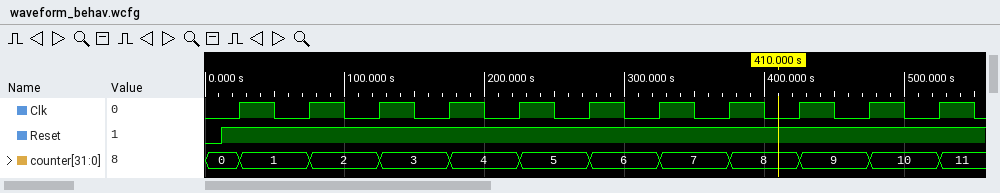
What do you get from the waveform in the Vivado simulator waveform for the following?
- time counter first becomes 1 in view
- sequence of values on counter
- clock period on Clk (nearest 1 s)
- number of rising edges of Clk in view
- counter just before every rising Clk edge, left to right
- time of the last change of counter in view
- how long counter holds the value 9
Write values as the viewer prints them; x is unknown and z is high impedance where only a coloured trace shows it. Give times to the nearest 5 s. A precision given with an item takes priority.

25 s
0, 1, 2, 3, 4, 5, 6, 7, 8, 9, 10, 11
50 s
11
0, 1, 2, 3, 4, 5, 6, 7, 8, 9, 10
525 s
50 s
